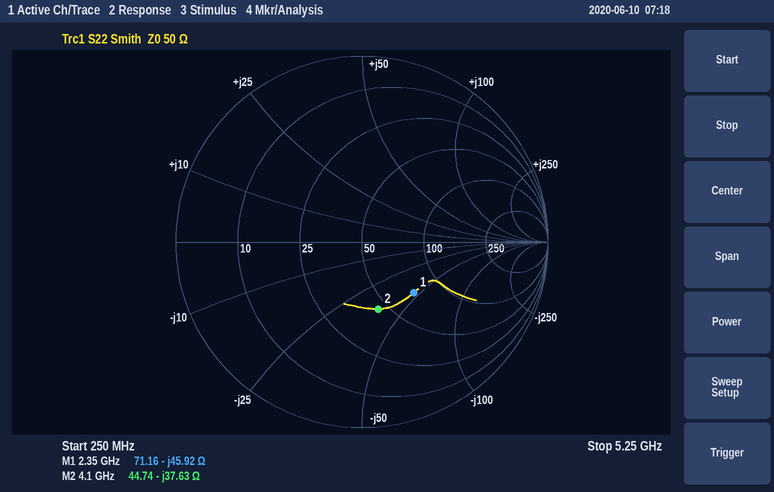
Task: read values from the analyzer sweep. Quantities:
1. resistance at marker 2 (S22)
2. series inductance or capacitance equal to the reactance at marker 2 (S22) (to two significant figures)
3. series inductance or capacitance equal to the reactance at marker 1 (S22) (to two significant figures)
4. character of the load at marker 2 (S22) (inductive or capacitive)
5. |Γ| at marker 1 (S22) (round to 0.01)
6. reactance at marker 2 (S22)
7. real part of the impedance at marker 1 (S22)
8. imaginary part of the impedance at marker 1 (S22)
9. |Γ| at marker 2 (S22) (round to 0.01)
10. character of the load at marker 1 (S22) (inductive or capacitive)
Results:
44.74 Ω
1.0 pF
1.5 pF
capacitive
0.39
-37.63 Ω
71.16 Ω
-45.92 Ω
0.37
capacitive
